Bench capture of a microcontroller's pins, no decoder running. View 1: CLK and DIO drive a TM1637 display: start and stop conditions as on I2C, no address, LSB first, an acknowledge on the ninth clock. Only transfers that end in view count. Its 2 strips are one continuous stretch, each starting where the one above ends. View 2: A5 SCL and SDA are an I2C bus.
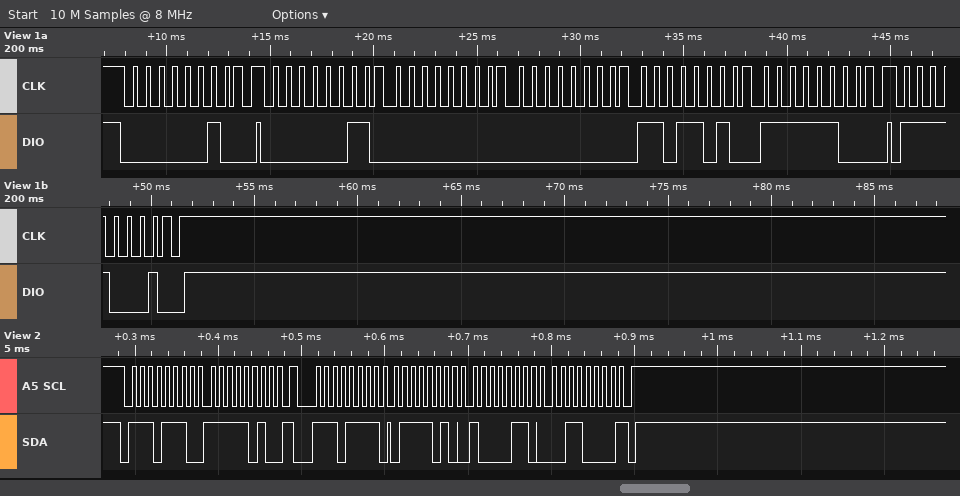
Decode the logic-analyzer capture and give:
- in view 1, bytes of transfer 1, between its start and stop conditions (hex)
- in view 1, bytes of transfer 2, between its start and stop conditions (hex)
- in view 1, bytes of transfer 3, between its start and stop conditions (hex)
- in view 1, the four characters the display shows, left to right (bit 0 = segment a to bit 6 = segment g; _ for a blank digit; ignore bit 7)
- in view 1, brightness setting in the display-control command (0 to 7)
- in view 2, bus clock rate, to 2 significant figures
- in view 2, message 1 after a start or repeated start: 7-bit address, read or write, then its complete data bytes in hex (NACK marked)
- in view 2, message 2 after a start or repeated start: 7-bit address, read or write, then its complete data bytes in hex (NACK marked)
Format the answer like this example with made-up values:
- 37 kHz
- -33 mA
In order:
- 40
- C0 00 00 5B 3F
- 8F
- __20
- 7
- 100 kHz
- 0x77 write: FA
- 0x77 read: 7A 86 30 NACK
